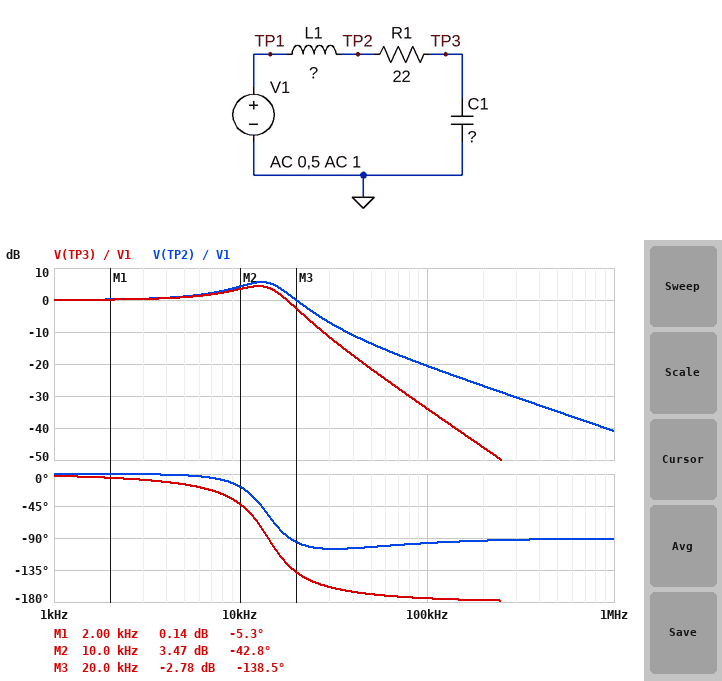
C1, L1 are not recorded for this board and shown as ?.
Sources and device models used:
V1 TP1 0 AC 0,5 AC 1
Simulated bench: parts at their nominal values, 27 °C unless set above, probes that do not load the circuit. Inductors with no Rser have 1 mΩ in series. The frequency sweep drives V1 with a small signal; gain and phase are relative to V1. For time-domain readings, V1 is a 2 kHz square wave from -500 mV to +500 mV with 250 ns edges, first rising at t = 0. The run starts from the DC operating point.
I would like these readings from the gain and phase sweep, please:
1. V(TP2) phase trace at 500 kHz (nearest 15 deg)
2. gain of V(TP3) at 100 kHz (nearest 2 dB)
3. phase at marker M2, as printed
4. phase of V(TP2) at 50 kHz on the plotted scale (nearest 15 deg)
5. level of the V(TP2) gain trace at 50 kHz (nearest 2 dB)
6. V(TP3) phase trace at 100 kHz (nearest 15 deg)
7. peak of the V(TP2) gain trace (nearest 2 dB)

-90 deg
-34 dB
-42.8 deg
-105 deg
-14 dB
-180 deg
6 dB
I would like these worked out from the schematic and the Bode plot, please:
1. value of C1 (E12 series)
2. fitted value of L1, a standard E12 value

330 nF
390 µH
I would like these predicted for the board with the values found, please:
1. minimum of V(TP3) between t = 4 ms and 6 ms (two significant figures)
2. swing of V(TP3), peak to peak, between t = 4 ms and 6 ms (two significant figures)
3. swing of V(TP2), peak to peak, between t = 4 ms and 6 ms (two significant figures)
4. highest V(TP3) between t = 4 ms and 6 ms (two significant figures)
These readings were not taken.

-850 mV
1.7 V
1.9 V
850 mV
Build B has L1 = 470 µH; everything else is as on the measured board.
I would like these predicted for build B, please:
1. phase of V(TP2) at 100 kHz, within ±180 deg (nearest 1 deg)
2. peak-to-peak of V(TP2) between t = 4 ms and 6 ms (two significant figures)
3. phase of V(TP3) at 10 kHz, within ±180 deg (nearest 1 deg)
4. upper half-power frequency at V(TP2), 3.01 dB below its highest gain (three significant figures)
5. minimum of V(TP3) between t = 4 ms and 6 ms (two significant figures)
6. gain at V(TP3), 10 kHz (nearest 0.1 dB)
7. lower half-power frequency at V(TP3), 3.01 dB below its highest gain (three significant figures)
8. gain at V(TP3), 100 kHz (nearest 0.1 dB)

-98 deg
1.9 V
-50 deg
15.5 kHz
-880 mV
4.5 dB
6.67 kHz
-35.6 dB
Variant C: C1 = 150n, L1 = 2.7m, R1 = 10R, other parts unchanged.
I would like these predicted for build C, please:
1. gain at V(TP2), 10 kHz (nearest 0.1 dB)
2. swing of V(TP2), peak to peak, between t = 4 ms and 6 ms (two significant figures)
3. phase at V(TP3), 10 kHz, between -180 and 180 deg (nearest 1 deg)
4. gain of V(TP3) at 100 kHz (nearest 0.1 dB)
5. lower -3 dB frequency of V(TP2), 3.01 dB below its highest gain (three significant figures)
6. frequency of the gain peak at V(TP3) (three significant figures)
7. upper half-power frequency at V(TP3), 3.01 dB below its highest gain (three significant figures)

4.4 dB
2.1 V
-171 deg
-44.0 dB
7.60 kHz
7.90 kHz
8.19 kHz
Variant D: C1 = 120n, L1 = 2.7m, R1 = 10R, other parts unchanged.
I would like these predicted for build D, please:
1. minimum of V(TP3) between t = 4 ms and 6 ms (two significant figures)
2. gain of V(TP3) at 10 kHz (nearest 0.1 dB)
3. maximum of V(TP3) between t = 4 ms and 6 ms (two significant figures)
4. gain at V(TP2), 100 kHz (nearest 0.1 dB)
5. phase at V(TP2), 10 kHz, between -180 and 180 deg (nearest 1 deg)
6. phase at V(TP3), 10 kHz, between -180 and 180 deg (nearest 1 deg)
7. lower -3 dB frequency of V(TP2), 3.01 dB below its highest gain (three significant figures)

-1.2 V
10.8 dB
1.2 V
-40.1 dB
-161 deg
-165 deg
8.53 kHz
